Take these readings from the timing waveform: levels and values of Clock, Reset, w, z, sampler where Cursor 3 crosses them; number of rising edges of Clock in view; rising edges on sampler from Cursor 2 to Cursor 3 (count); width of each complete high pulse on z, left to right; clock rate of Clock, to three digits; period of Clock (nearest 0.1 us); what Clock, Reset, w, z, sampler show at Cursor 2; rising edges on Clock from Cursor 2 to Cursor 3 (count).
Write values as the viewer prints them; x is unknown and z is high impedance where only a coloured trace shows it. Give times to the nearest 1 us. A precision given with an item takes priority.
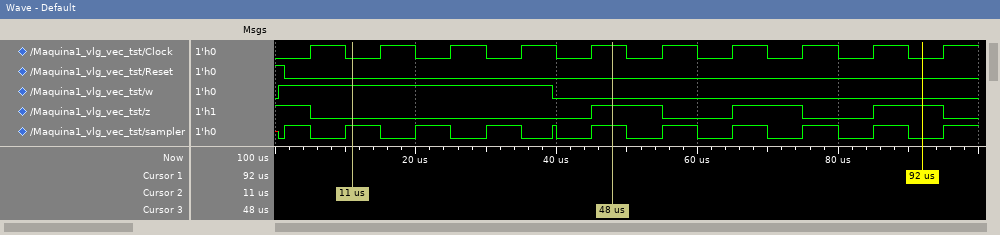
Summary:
Clock=1, Reset=0, w=0, z=1, sampler=1
10
4
10 us, 10 us, 10 us
100 kHz
10 us
Clock=0, Reset=0, w=1, z=0, sampler=1
4
